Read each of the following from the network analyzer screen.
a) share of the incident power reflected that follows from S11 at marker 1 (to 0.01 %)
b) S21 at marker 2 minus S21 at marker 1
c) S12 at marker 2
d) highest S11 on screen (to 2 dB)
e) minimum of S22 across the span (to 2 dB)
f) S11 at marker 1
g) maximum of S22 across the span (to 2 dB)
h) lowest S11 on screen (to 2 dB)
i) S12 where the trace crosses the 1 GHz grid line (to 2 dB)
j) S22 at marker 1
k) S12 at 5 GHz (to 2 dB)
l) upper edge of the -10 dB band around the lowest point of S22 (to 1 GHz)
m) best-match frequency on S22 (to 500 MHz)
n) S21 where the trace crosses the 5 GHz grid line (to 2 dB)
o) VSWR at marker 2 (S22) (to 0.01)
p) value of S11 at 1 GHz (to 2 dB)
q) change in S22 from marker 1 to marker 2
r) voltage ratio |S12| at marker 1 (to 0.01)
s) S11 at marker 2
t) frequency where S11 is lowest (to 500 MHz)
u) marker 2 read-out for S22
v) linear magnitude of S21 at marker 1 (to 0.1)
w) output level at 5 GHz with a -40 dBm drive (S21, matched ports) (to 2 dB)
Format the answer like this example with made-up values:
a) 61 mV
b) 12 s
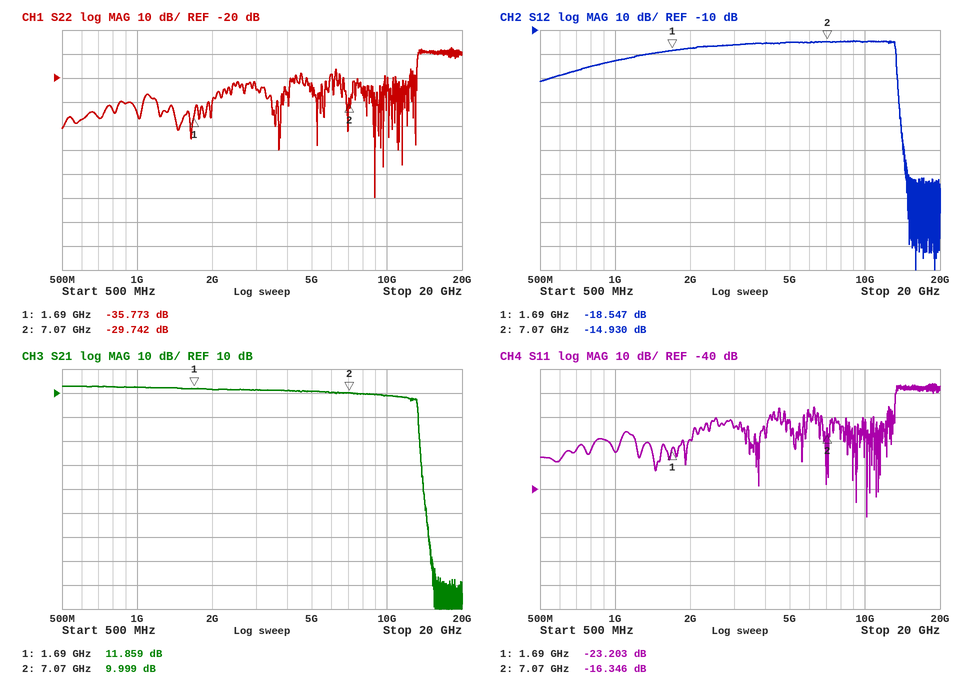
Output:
a) 0.48 %
b) -1.860 dB
c) -14.930 dB
d) 4 dB
e) -70 dB
f) -23.203 dB
g) -8 dB
h) -52 dB
i) -22 dB
j) -35.773 dB
k) -16 dB
l) 13 GHz
m) 9.0 GHz
n) 10 dB
o) 1.07
p) -24 dB
q) 6.031 dB
r) 0.12
s) -16.346 dB
t) 10.0 GHz
u) -29.742 dB
v) 3.9
w) -30 dBm
